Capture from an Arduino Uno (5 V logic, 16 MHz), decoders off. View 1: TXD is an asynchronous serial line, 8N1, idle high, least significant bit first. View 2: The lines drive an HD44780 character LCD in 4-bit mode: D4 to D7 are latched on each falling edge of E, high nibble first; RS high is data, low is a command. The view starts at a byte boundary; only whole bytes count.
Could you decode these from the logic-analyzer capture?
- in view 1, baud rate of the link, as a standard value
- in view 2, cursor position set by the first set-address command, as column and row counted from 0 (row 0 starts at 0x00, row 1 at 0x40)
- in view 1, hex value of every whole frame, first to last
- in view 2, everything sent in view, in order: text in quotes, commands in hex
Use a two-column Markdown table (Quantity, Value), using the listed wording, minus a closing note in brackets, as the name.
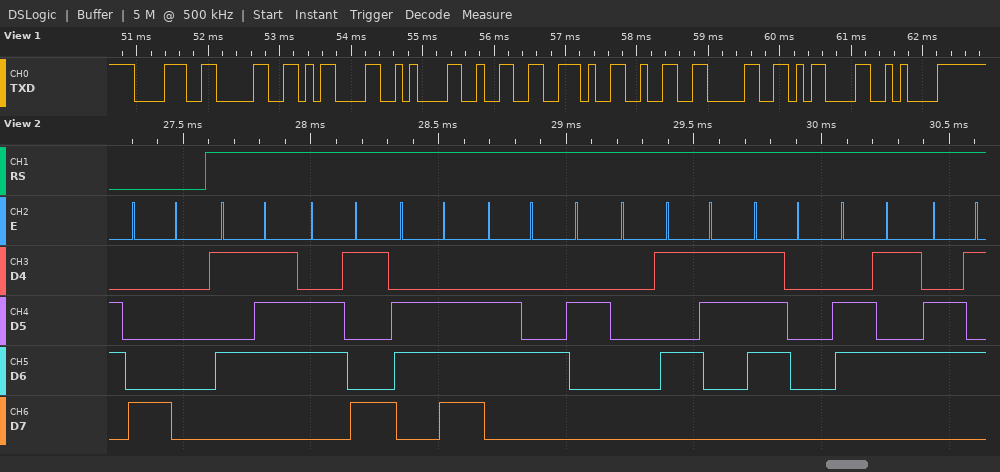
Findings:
| Quantity | Value |
|---|---|
| in view 1, baud rate of the link, as a standard value | 9600 baud |
| in view 2, cursor position set by the first set-address command, as column and row counted from 0 | column 0, row 0 |
| in view 1, hex value of every whole frame, first to last | 0x38 0x30 0x0D 0x0A 0x32 0x2E 0x32 0x30 0x0D 0x0A |
| in view 2, everything sent in view, in order: text in quotes, commands in hex | 0x80 "Wind Spee" |
